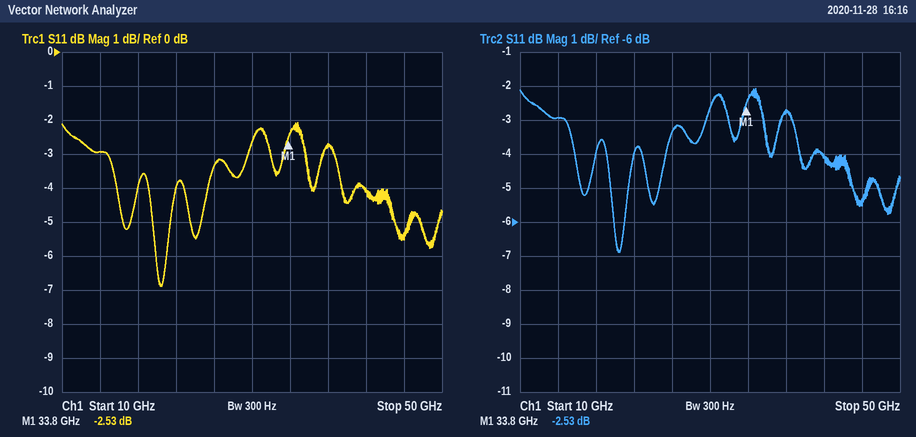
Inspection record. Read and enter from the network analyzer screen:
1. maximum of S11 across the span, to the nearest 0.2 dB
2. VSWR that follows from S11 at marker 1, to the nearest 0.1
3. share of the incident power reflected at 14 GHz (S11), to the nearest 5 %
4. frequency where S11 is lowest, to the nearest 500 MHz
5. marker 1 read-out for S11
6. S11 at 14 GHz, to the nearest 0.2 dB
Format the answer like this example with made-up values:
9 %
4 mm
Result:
-2.0 dB
6.9
50 %
20.5 GHz
-2.53 dB
-3.0 dB
